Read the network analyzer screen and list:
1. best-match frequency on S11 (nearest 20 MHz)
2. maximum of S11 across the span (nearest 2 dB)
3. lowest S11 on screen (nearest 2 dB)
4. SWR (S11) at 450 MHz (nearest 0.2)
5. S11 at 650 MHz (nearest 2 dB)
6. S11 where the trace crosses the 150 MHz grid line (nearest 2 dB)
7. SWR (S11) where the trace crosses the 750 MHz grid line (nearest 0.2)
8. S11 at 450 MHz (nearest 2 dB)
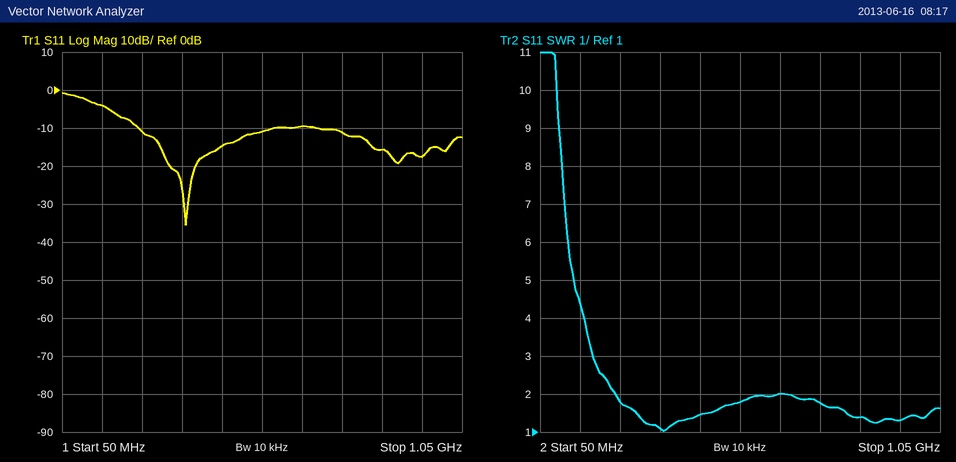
360 MHz
0 dB
-36 dB
1.4
-10 dB
-4 dB
1.8
-14 dB
